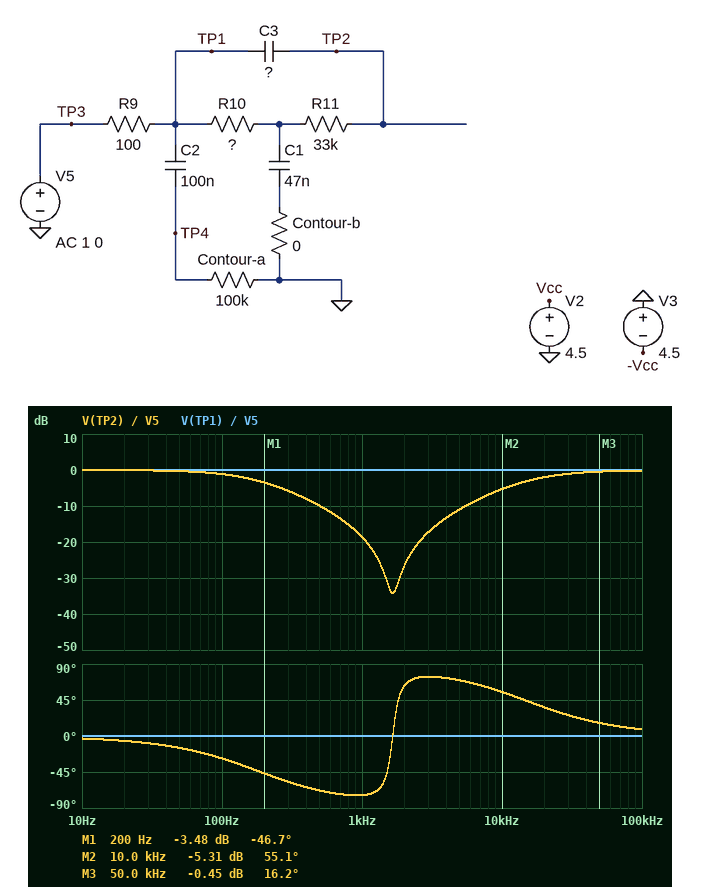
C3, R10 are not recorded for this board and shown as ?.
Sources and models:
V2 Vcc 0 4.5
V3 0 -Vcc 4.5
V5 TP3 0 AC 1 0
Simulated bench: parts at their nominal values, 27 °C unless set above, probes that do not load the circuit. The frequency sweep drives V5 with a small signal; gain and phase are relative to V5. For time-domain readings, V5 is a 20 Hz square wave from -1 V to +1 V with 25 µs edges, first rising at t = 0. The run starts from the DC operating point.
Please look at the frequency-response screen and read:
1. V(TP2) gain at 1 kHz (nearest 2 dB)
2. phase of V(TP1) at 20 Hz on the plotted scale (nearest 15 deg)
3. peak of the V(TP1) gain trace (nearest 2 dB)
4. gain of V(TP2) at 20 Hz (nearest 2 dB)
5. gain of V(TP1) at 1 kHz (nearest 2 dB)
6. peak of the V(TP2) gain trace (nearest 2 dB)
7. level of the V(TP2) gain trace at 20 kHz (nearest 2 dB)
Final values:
-18 dB
0 deg
0 dB
0 dB
0 dB
0 dB
-2 dB
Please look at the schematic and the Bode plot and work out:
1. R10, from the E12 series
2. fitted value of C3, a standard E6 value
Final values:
18 kΩ
330 pF
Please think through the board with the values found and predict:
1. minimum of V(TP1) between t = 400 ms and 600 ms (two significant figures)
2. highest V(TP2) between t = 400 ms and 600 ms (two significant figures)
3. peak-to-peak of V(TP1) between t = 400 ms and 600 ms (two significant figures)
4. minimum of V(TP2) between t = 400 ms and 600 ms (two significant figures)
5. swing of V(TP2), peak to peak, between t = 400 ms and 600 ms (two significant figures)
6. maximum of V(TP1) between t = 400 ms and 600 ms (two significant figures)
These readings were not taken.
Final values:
-1.0 V
1.0 V
2.0 V
-1.0 V
2.0 V
1.0 V
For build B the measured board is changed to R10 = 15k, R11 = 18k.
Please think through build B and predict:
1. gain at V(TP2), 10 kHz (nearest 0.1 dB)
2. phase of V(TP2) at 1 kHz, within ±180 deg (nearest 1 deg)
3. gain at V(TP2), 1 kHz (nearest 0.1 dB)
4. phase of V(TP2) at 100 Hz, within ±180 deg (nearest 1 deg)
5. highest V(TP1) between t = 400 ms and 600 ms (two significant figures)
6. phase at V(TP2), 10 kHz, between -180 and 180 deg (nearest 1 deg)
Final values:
-9.8 dB
-75 deg
-14.8 dB
-24 deg
1.0 V
68 deg
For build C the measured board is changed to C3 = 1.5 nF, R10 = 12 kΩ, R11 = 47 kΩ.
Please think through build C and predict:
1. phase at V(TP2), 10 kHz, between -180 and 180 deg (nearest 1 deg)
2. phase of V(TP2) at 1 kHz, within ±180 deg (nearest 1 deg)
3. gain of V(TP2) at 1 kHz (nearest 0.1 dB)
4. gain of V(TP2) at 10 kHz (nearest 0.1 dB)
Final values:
13 deg
38 deg
-14.4 dB
-0.4 dB
